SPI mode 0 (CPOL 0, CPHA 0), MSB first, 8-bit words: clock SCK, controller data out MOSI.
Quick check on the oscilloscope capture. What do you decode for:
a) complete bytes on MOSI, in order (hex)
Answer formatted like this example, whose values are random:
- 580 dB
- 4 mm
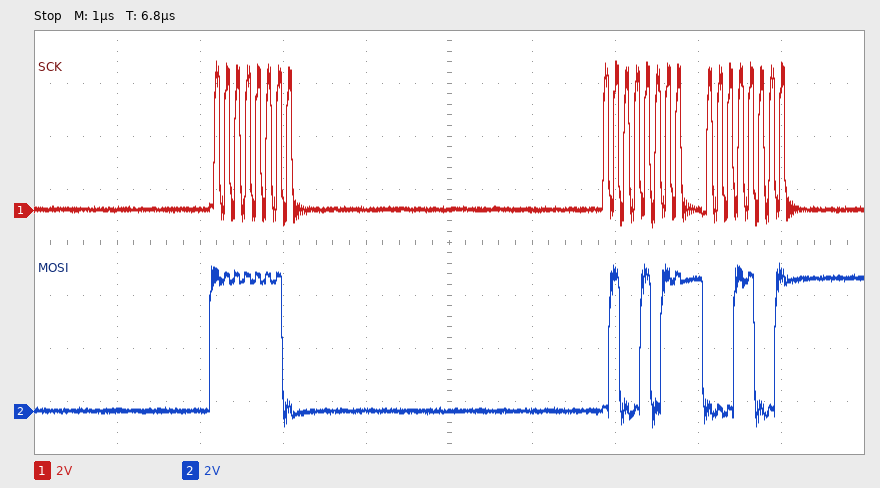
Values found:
- FE 4B 19
